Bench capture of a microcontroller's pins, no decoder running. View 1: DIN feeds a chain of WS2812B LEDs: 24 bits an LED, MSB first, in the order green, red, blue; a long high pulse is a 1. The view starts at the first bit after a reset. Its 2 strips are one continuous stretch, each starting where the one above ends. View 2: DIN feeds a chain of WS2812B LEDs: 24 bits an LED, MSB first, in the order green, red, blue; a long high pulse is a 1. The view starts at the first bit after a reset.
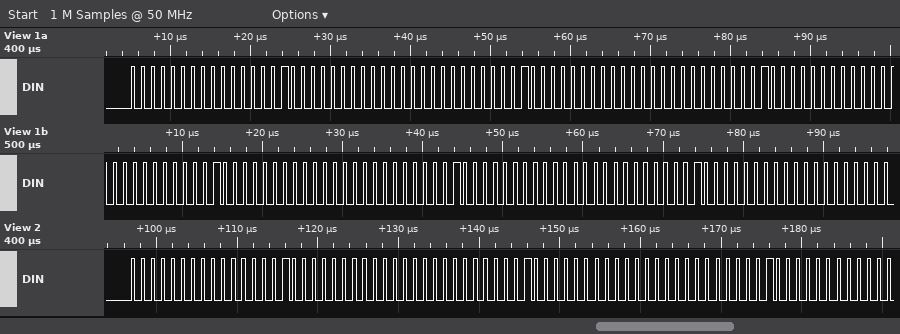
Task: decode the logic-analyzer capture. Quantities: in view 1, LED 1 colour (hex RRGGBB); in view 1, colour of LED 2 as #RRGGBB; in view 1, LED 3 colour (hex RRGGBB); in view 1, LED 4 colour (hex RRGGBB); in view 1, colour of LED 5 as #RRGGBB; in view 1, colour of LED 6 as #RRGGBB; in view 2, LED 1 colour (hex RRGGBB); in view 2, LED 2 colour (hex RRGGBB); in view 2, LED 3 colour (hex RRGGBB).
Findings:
#010000
#010000
#010000
#010000
#010000
#010000
#010000
#010000
#010000
